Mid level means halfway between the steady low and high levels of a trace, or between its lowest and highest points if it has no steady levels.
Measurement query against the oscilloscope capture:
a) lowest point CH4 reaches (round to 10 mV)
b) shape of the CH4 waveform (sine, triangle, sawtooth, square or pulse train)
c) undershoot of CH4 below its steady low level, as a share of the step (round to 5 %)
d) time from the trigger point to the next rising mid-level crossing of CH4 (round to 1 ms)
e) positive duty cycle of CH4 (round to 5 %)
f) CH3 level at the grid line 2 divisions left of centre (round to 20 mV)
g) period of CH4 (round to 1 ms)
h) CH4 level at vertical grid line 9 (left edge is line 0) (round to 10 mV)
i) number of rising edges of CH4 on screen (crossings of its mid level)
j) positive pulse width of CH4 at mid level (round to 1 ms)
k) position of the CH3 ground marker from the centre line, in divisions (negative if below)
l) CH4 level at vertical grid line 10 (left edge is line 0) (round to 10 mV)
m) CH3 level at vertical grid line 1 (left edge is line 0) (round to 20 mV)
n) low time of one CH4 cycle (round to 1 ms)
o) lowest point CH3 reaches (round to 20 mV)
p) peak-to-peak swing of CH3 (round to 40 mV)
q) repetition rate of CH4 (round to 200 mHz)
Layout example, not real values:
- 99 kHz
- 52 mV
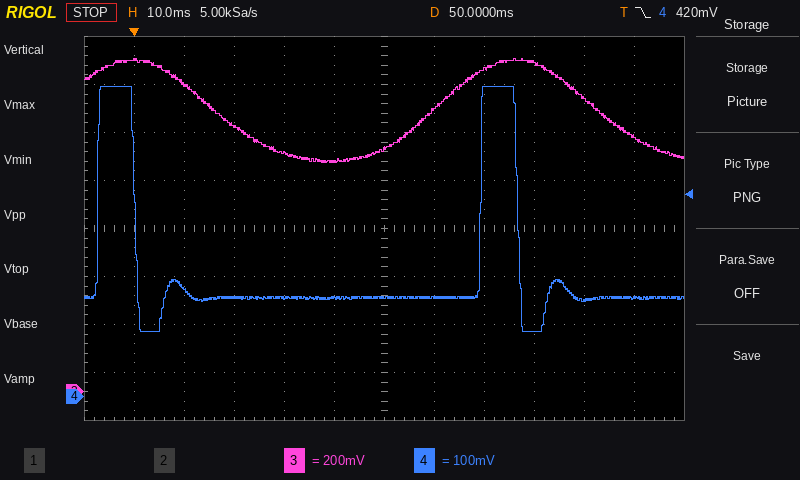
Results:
- 140 mV
- pulse train
- 15 %
- 69 ms
- 10 %
- 1.00 V
- 77 ms
- 140 mV
- 2
- 7 ms
- -3.4 div
- 200 mV
- 1.38 V
- 69 ms
- 960 mV
- 440 mV
- 13.0 Hz
